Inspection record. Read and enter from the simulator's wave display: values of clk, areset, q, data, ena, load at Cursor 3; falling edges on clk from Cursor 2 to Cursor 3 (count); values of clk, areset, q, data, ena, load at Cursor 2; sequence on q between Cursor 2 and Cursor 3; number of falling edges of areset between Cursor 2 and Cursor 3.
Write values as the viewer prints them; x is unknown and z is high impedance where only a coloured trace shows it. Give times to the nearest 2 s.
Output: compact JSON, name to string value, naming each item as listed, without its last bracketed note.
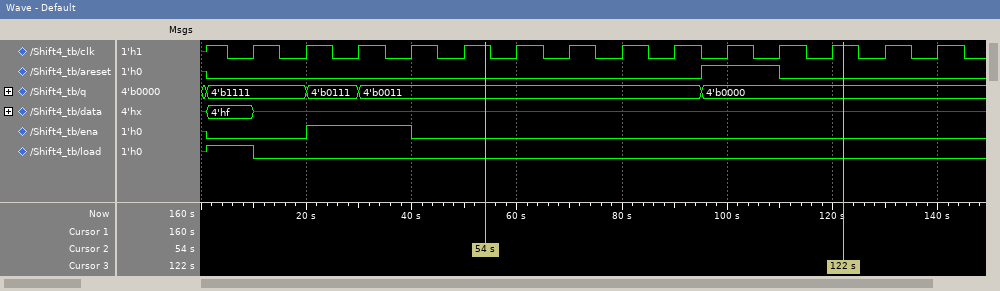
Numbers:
{"values of clk, areset, q, data, ena, load at Cursor 3": "clk=1, areset=0, q=4'b0000, data=x, ena=0, load=0", "falling edges on clk from Cursor 2 to Cursor 3": "7", "values of clk, areset, q, data, ena, load at Cursor 2": "clk=1, areset=0, q=4'b0011, data=x, ena=0, load=0", "sequence on q between Cursor 2 and Cursor 3": "4'b0011, 4'b0000", "number of falling edges of areset between Cursor 2 and Cursor 3": "1"}
